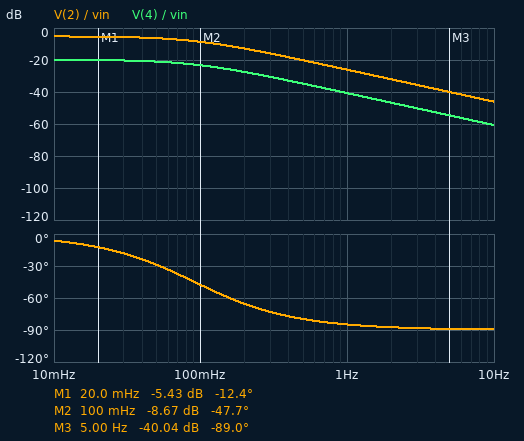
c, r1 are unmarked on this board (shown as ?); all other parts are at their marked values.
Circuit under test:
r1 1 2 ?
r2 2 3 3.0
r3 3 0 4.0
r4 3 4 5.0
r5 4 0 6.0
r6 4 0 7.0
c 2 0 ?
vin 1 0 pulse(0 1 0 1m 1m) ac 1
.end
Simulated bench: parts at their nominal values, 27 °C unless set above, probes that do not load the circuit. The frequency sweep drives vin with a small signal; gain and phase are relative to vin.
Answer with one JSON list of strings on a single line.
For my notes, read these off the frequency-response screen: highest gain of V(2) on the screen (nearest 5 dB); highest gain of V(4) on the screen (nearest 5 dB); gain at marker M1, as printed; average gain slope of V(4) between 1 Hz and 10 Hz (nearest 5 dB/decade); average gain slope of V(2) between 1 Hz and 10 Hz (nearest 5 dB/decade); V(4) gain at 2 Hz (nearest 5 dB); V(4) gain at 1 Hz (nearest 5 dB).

["-5 dB", "-20 dB", "-5.43 dB", "-20 dB/decade", "-20 dB/decade", "-45 dB", "-40 dB"]
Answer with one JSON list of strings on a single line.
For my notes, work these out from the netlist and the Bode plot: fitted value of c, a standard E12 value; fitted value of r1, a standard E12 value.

["680 mF", "4.7 Ω"]
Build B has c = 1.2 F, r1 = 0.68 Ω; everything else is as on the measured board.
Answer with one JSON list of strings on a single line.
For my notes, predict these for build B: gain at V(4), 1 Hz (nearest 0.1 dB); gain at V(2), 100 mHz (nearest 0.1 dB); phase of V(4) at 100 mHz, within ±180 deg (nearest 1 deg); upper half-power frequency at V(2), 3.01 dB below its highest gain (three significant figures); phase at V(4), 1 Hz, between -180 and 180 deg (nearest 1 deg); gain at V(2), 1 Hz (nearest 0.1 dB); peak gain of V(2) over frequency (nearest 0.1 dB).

["-29.0 dB", "-1.8 dB", "-25 deg", "218 mHz", "-78 deg", "-14.4 dB", "-1.0 dB"]
